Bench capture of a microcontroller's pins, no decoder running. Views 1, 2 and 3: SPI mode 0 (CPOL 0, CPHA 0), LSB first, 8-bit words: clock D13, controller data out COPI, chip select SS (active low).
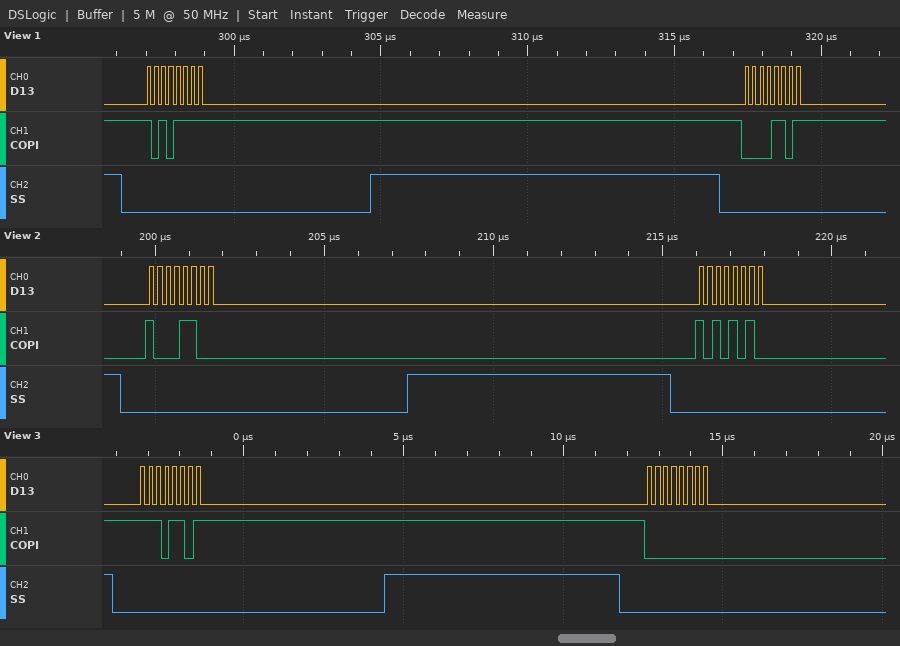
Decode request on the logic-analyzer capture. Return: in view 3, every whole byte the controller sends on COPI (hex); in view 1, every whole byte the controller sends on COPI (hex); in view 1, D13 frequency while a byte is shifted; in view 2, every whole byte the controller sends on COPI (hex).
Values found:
0xB7 0x00
0xF5 0xB0
4 MHz
31 55
